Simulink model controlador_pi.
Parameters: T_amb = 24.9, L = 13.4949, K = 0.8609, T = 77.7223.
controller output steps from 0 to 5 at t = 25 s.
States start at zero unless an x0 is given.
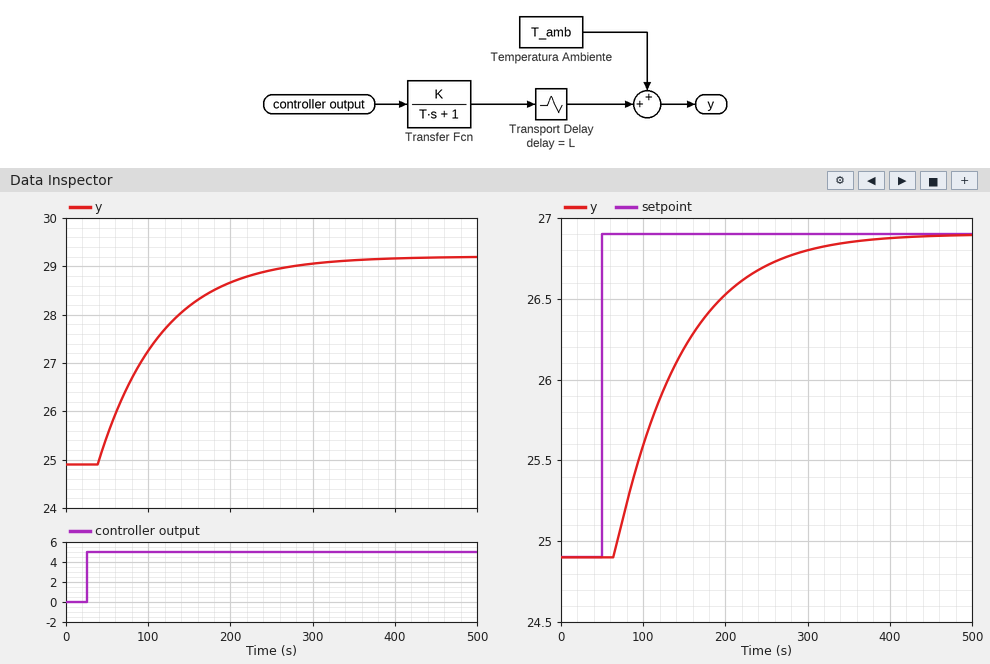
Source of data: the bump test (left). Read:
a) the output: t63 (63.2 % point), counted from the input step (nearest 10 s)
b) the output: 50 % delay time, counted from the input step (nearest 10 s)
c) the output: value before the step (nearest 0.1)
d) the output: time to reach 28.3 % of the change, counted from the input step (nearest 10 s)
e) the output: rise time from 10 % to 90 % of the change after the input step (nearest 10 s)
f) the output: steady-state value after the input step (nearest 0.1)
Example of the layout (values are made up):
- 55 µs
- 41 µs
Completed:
- 90 s
- 70 s
- 24.9
- 40 s
- 170 s
- 29.2
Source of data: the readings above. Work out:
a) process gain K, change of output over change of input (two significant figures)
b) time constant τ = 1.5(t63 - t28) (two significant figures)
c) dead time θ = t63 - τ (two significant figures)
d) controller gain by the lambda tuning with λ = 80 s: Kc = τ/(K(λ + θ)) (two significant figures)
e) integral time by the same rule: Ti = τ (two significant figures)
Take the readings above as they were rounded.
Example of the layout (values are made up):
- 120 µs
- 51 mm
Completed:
- 0.86
- 75 s
- 15 s
- 0.92
- 75 s
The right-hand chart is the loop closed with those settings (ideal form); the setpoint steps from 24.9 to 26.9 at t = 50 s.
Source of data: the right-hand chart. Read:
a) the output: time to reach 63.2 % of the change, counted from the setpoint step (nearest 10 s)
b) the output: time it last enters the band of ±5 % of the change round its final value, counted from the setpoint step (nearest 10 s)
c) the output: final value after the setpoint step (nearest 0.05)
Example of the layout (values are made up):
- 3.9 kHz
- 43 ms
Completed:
- 100 s
- 250 s
- 26.90
